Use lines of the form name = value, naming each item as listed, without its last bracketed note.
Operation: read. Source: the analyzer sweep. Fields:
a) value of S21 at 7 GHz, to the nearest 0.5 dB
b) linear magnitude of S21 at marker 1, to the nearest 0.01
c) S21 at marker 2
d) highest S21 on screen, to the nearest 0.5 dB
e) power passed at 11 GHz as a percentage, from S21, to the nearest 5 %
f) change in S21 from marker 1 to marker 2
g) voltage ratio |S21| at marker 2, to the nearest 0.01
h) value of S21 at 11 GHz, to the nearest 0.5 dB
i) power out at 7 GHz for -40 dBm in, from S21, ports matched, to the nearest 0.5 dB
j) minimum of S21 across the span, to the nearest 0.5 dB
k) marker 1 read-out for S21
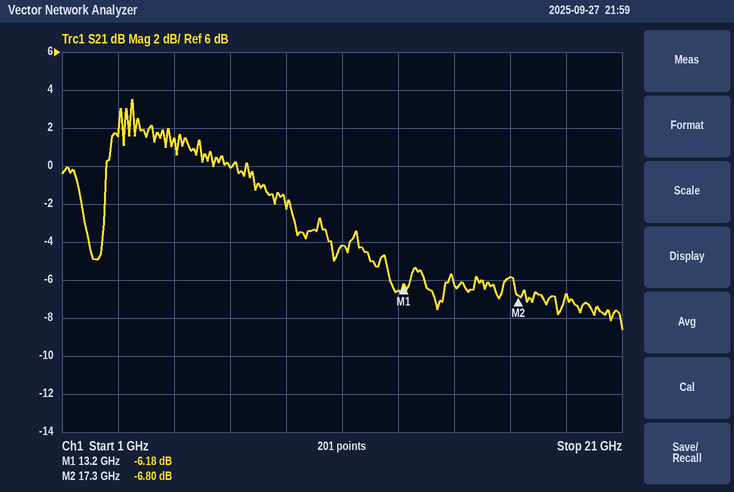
value of S21 at 7 GHz, to the nearest 0.5 dB = 0.0 dB
linear magnitude of S21 at marker 1, to the nearest 0.01 = 0.49
S21 at marker 2 = -6.80 dB
highest S21 on screen, to the nearest 0.5 dB = 3.5 dB
power passed at 11 GHz as a percentage, from S21, to the nearest 5 % = 40 %
change in S21 from marker 1 to marker 2 = -0.62 dB
voltage ratio |S21| at marker 2, to the nearest 0.01 = 0.46
value of S21 at 11 GHz, to the nearest 0.5 dB = -4.0 dB
power out at 7 GHz for -40 dBm in, from S21, ports matched, to the nearest 0.5 dB = -40.0 dBm
minimum of S21 across the span, to the nearest 0.5 dB = -8.5 dB
marker 1 read-out for S21 = -6.18 dB
